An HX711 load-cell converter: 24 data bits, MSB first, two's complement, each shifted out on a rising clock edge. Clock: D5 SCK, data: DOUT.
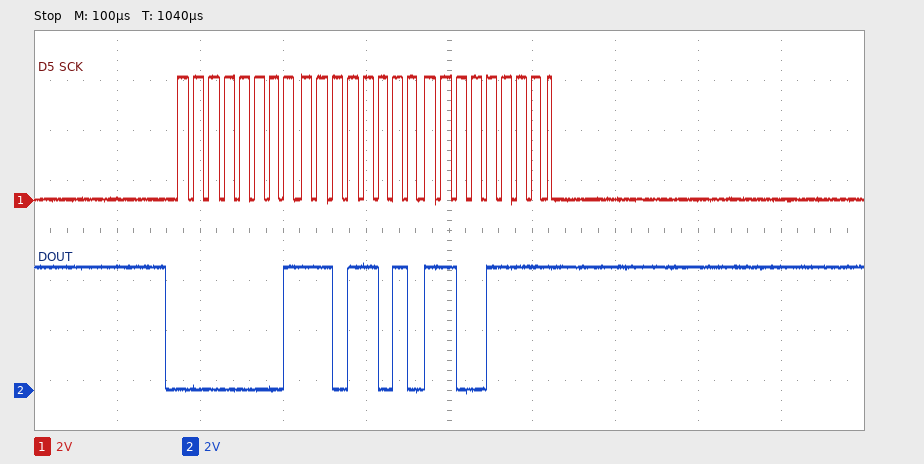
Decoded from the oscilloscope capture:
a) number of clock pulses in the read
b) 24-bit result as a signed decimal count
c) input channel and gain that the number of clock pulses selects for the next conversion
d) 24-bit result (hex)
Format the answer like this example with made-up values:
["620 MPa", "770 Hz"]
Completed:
["25", "121551", "channel A, gain 128", "0x01DACF"]
